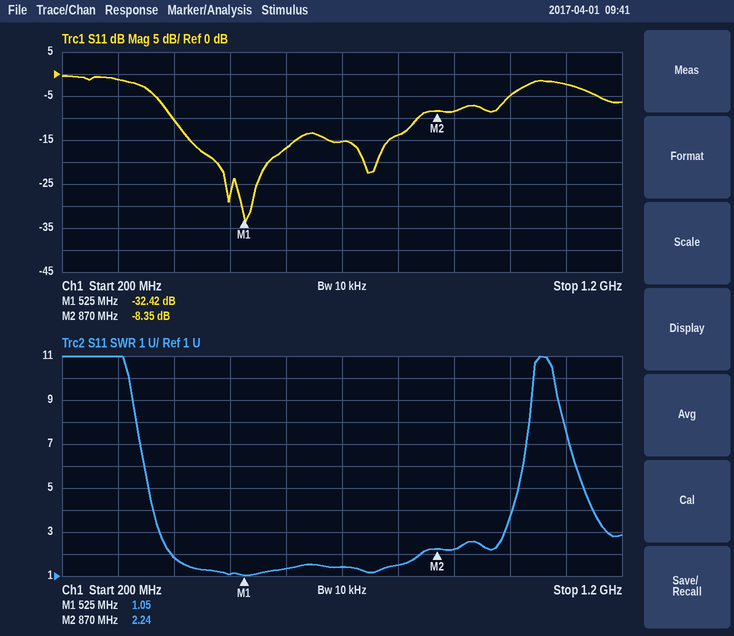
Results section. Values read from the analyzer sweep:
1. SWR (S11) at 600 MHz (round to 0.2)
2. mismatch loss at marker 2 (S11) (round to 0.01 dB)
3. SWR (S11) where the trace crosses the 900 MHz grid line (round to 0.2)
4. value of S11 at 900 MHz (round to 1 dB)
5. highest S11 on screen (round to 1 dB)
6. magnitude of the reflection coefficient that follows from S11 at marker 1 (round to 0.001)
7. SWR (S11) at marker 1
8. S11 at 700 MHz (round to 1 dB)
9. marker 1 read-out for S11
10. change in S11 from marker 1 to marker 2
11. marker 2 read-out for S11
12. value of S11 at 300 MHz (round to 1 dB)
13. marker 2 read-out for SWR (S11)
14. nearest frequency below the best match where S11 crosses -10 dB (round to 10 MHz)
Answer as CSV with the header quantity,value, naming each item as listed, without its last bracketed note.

quantity,value
SWR (S11) at 600 MHz,1.4
mismatch loss at marker 2 (S11),0.69 dB
SWR (S11) where the trace crosses the 900 MHz grid line,2.2
value of S11 at 900 MHz,-8 dB
highest S11 on screen,0 dB
magnitude of the reflection coefficient that follows from S11 at marker 1,0.024
SWR (S11) at marker 1,1.05
S11 at 700 MHz,-15 dB
marker 1 read-out for S11,-32.42 dB
change in S11 from marker 1 to marker 2,24.07 dB
marker 2 read-out for S11,-8.35 dB
value of S11 at 300 MHz,-1 dB
marker 2 read-out for SWR,2.24
nearest frequency below the best match where S11 crosses -10 dB,400 MHz
